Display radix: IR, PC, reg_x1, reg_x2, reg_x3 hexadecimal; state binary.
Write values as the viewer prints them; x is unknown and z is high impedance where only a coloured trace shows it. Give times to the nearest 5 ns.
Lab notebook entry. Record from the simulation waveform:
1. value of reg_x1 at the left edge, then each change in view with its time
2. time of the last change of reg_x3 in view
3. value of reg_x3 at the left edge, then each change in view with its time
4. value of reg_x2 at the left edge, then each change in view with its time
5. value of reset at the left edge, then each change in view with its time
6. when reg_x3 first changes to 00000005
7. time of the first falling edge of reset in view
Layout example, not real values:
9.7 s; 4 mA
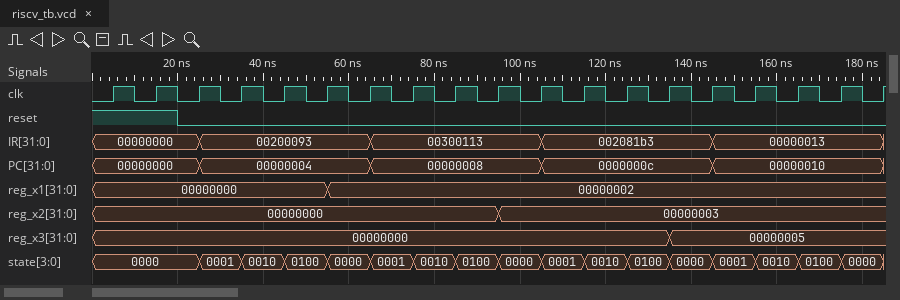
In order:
00000000, 00000002 at 55 ns; 135 ns; 00000000, 00000005 at 135 ns; 00000000, 00000003 at 95 ns; 1, 0 at 20 ns; 135 ns; 20 ns
